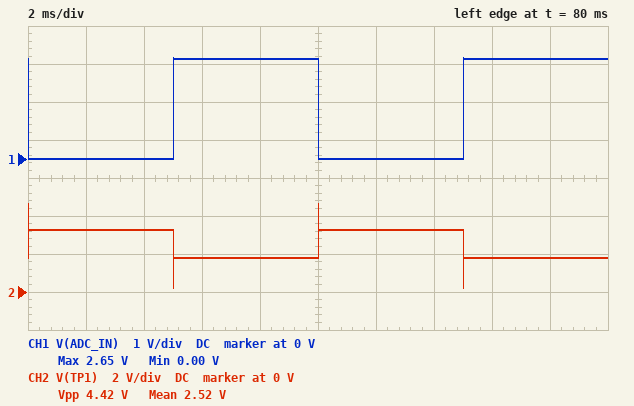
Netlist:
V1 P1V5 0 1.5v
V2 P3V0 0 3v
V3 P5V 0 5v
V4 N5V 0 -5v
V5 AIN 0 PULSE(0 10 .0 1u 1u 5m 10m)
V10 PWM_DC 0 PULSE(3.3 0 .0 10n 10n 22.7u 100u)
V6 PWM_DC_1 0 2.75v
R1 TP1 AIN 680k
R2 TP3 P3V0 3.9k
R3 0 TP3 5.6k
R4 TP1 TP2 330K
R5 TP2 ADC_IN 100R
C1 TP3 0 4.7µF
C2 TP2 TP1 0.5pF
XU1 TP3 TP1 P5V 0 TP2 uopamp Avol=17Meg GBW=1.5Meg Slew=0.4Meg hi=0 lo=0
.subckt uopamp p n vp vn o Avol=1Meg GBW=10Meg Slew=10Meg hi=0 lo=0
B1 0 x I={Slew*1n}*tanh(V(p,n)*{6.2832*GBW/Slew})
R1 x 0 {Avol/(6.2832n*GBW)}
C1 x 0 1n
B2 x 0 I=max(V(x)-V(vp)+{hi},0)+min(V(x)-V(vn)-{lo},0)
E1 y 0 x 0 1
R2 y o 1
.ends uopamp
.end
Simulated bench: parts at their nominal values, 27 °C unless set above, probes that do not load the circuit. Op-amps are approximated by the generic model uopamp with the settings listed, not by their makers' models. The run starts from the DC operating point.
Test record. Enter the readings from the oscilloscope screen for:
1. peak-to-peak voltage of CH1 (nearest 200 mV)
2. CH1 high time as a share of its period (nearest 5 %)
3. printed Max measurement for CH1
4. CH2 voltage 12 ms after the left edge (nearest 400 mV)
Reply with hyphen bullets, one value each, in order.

- 2.6 V
- 50 %
- 2.65 V
- 3.2 V
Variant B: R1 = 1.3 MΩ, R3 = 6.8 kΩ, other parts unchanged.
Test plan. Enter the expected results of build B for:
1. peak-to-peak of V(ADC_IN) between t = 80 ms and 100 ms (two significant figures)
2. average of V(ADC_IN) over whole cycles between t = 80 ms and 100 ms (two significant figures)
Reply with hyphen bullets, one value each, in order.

- 2.4 V
- 1.2 V
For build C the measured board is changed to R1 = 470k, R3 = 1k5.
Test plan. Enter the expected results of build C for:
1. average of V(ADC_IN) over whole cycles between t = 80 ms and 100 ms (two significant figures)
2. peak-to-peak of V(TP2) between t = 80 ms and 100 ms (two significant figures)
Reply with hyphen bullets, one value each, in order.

- 710 mV
- 1.4 V
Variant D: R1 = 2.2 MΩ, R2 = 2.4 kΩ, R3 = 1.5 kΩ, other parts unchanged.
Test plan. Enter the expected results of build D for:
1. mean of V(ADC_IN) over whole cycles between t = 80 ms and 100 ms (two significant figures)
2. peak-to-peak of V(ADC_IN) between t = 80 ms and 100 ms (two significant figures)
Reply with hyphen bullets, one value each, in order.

- 660 mV
- 1.3 V
